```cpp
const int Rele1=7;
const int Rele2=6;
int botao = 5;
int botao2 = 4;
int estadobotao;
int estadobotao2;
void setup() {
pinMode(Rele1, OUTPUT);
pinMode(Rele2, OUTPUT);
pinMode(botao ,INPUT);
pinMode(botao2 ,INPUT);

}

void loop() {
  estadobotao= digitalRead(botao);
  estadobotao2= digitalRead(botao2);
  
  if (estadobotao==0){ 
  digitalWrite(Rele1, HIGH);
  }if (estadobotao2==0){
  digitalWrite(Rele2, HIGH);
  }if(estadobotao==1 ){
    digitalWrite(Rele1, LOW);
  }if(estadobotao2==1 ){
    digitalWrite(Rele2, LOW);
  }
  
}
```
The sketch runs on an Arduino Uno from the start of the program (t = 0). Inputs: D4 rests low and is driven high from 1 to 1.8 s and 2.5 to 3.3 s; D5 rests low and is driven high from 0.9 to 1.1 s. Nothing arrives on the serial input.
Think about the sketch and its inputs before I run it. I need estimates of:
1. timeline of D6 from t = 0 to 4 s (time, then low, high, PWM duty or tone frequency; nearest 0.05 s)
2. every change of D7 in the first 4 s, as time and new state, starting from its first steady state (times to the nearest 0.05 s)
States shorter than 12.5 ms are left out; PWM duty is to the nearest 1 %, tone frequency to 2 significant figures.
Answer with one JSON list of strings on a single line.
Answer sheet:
["0 s high; 1 s low; 1.8 s high; 2.5 s low; 3.3 s high", "0 s high; 0.9 s low; 1.1 s high"]
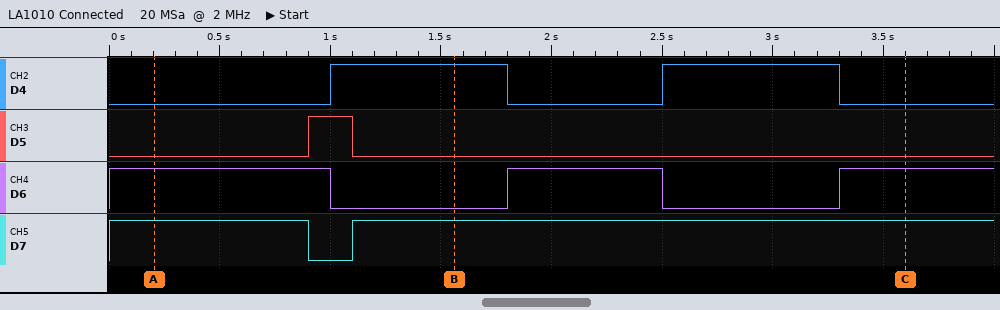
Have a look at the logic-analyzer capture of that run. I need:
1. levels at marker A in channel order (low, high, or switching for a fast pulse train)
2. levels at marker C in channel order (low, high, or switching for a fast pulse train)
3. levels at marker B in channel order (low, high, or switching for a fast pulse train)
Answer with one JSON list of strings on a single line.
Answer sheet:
["D4 low, D5 low, D6 high, D7 high", "D4 low, D5 low, D6 high, D7 high", "D4 high, D5 low, D6 low, D7 high"]
